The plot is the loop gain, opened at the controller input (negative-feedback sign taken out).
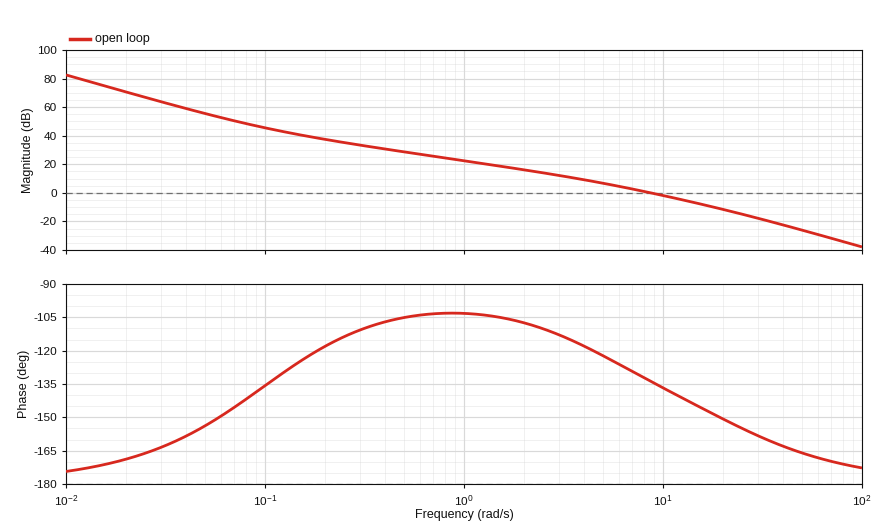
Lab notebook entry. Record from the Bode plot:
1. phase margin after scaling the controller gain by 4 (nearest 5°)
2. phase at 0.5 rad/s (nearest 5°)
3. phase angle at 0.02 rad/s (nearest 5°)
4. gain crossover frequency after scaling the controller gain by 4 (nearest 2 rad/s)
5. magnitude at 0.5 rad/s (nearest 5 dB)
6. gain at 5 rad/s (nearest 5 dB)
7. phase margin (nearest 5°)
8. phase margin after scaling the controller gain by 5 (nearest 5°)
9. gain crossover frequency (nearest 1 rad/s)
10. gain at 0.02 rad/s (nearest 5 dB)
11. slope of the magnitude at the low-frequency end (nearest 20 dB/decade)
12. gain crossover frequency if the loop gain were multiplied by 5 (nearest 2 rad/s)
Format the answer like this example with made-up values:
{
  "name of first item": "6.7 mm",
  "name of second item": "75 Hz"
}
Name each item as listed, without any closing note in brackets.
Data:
{
  "phase margin after scaling the controller gain by 4": "30°",
  "phase at 0.5 rad/s": "-105°",
  "phase angle at 0.02 rad/s": "-170°",
  "gain crossover frequency after scaling the controller gain by 4": "20 rad/s",
  "magnitude at 0.5 rad/s": "30 dB",
  "gain at 5 rad/s": "5 dB",
  "phase margin": "45°",
  "phase margin after scaling the controller gain by 5": "25°",
  "gain crossover frequency": "9 rad/s",
  "gain at 0.02 rad/s": "70 dB",
  "slope of the magnitude at the low-frequency end": "-40 dB/decade",
  "gain crossover frequency if the loop gain were multiplied by 5": "24 rad/s"
}
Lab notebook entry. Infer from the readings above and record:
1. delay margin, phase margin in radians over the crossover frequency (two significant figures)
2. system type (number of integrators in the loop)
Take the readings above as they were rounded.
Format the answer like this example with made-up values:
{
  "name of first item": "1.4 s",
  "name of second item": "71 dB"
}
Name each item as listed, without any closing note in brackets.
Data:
{
  "delay margin, phase margin in radians over the crossover frequency": "0.087 s",
  "system type": "2"
}
